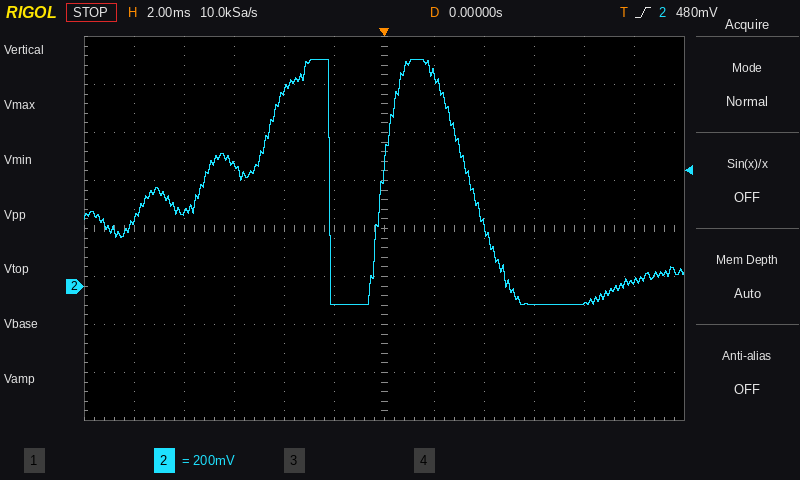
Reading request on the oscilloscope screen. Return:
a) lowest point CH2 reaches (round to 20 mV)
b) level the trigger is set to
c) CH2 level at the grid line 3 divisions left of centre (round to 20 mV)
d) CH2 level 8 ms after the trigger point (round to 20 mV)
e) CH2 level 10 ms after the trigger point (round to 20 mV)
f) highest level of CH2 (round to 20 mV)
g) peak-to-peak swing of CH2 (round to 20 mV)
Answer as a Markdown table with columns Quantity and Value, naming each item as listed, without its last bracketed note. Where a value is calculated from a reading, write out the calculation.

| Quantity | Value |
|---|---|
| lowest point CH2 reaches | -80 mV |
| level the trigger is set to | 480 mV |
| CH2 level at the grid line 3 divisions left of centre | 500 mV |
| CH2 level 8 ms after the trigger point | -80 mV |
| CH2 level 10 ms after the trigger point | 20 mV |
| highest level of CH2 | 940 mV |
| peak-to-peak swing of CH2 | 940 mV − (-80 mV) = 1.02 V |
